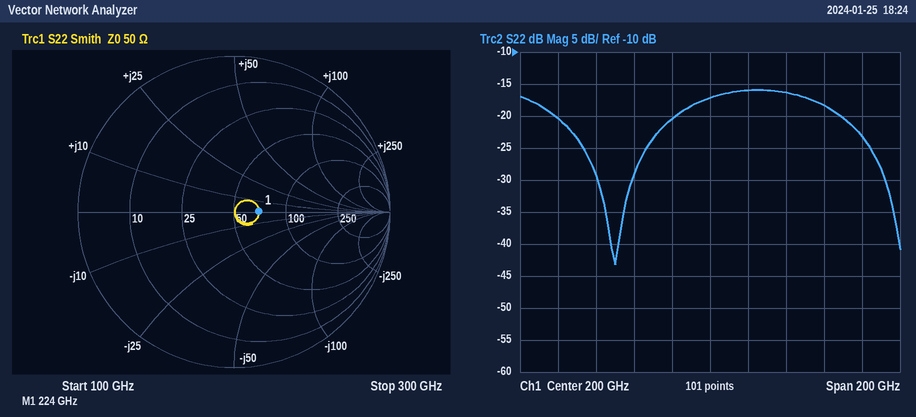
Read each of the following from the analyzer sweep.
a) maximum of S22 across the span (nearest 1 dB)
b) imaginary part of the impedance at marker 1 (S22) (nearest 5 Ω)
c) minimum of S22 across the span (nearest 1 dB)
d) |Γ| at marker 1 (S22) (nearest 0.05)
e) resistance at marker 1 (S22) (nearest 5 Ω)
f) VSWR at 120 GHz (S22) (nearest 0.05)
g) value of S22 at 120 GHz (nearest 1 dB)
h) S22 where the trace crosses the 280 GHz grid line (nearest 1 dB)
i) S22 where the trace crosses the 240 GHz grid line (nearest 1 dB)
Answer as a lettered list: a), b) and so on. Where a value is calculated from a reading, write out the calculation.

a) -16 dB
b) 0 Ω
c) -43 dB
d) 0.15
e) 70 Ω
f) |Γ| = 10^(-20/20) = 0.1000; VSWR = (1 + 0.1000)/(1 − 0.1000) ≈ 1.22, so 1.20 to the nearest 0.05
g) -20 dB
h) -23 dB
i) -16 dB
